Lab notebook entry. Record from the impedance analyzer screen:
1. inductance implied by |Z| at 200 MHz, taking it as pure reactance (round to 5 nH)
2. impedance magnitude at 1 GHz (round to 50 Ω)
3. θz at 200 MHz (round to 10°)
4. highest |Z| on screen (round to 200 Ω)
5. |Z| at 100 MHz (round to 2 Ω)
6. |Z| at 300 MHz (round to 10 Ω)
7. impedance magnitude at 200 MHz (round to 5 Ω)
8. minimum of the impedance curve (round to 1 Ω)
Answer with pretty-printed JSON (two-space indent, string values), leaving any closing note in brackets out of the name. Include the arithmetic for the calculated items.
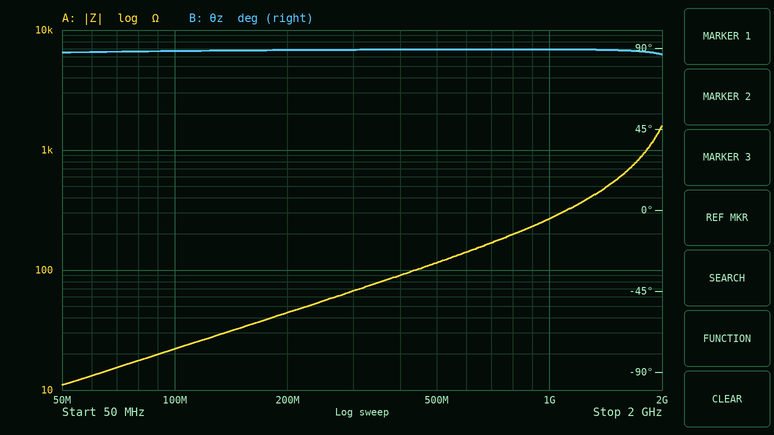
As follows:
{
  "inductance implied by |Z| at 200 MHz, taking it as pure reactance": "L = 45 Ω/(2π × 200 MHz) ≈ 35.8 nH, so 35 nH to the nearest 5 nH",
  "impedance magnitude at 1 GHz": "250 Ω",
  "θz at 200 MHz": "90°",
  "highest |Z| on screen": "1.6 kΩ",
  "|Z| at 100 MHz": "22 Ω",
  "|Z| at 300 MHz": "70 Ω",
  "impedance magnitude at 200 MHz": "45 Ω",
  "minimum of the impedance curve": "11 Ω"
}
